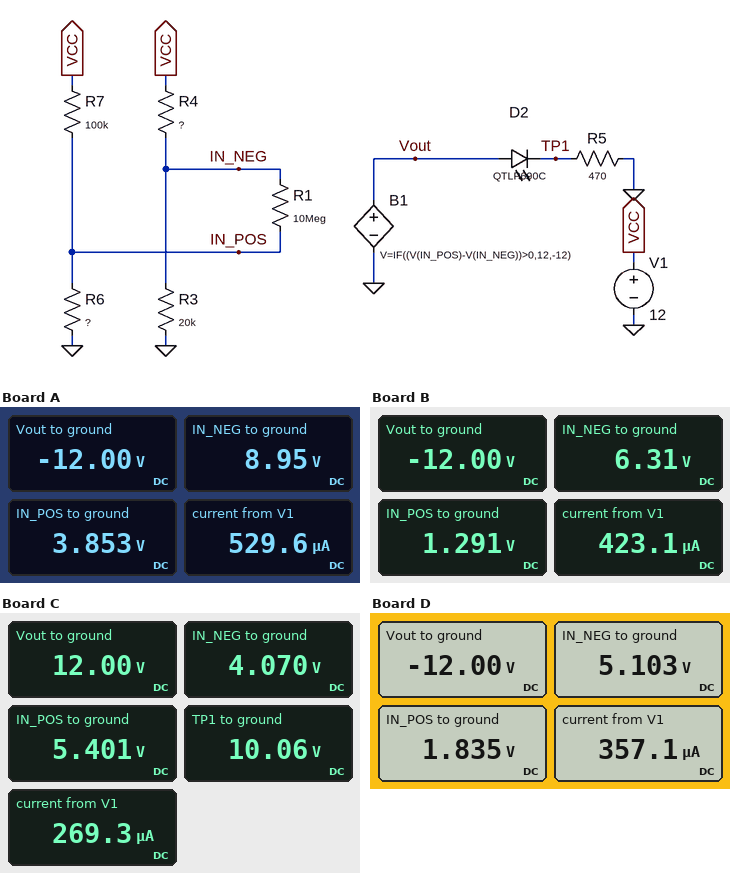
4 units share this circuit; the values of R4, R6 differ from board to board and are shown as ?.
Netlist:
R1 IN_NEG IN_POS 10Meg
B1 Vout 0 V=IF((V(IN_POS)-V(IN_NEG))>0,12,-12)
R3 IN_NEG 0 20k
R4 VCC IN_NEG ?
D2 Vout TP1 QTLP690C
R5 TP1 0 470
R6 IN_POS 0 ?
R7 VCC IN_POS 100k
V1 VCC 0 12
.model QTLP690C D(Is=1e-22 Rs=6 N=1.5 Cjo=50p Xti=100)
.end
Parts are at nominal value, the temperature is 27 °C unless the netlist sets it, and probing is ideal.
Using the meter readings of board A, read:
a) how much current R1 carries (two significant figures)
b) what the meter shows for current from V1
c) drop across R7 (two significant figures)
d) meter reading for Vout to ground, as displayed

510 nA
529.6 µA
8.1 V
-12.00 V
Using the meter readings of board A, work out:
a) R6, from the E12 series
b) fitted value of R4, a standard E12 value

47 kΩ
6.8 kΩ
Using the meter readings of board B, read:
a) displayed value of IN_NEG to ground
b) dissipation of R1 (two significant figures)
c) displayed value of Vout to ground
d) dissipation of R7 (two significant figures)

6.31 V
2.5 µW
-12.00 V
1.1 mW
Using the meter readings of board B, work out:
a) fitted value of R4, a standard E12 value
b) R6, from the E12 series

18 kΩ
12 kΩ
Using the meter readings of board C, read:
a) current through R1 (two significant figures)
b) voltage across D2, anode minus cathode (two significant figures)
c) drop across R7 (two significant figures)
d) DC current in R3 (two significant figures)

130 nA
1.9 V
6.6 V
200 µA
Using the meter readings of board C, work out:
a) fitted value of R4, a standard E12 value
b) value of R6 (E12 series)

39 kΩ
82 kΩ
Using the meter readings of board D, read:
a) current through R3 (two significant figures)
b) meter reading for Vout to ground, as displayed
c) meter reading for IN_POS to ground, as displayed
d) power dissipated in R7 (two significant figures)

260 µA
-12.00 V
1.835 V
1.0 mW
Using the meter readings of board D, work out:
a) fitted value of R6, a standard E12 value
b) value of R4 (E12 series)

18 kΩ
27 kΩ
